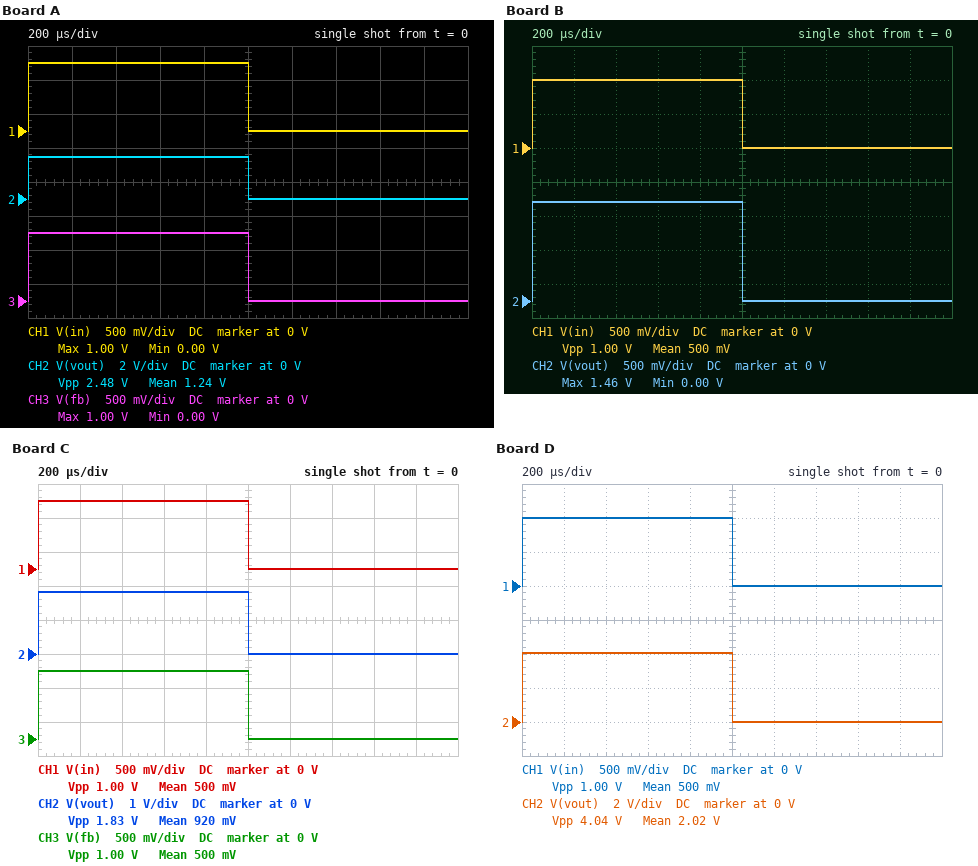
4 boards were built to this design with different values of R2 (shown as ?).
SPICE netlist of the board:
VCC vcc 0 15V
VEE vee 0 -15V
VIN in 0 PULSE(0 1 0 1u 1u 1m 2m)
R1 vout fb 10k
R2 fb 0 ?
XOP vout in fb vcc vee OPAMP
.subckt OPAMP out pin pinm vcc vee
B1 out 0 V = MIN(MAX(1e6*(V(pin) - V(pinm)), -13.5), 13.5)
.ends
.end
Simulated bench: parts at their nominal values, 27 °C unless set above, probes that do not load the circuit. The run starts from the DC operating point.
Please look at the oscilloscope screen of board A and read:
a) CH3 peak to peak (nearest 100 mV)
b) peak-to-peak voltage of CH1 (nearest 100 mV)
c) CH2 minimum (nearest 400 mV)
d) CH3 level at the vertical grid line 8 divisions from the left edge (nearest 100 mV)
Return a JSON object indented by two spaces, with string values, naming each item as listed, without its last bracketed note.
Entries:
{
  "CH3 peak to peak": "1.0 V",
  "peak-to-peak voltage of CH1": "1.0 V",
  "CH2 minimum": "0 V",
  "CH3 level at the vertical grid line 8 divisions from the left edge": "0 V"
}
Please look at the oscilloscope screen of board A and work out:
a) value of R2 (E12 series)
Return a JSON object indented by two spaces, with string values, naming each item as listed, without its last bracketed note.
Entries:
{
  "value of R2": "6.8 kΩ"
}
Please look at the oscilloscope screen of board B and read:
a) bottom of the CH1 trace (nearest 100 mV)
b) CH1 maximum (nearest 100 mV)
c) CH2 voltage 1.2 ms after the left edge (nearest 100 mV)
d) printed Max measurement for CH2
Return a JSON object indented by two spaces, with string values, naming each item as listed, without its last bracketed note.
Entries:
{
  "bottom of the CH1 trace": "0 V",
  "CH1 maximum": "1.0 V",
  "CH2 voltage 1.2 ms after the left edge": "0 V",
  "printed Max measurement for CH2": "1.46 V"
}
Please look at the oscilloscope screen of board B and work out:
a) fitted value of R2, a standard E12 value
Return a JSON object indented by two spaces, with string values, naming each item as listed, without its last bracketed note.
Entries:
{
  "fitted value of R2, a standard E12 value": "22 kΩ"
}
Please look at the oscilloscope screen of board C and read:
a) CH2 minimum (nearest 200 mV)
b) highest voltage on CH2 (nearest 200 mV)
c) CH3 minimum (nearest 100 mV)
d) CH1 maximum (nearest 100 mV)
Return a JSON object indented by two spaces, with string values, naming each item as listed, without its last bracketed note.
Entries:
{
  "CH2 minimum": "0 V",
  "highest voltage on CH2": "1.8 V",
  "CH3 minimum": "0 V",
  "CH1 maximum": "1.0 V"
}
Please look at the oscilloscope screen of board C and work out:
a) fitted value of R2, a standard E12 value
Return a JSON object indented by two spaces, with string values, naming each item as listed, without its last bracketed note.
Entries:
{
  "fitted value of R2, a standard E12 value": "12 kΩ"
}
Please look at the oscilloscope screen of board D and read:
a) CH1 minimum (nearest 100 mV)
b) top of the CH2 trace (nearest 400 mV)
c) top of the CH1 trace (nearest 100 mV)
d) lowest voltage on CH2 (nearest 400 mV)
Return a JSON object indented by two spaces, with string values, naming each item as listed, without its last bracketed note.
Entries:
{
  "CH1 minimum": "0 V",
  "top of the CH2 trace": "4.0 V",
  "top of the CH1 trace": "1.0 V",
  "lowest voltage on CH2": "0 V"
}
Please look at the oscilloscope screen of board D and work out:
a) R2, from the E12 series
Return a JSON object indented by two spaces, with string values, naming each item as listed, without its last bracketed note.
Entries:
{
  "R2, from the E12 series": "3.3 kΩ"
}
